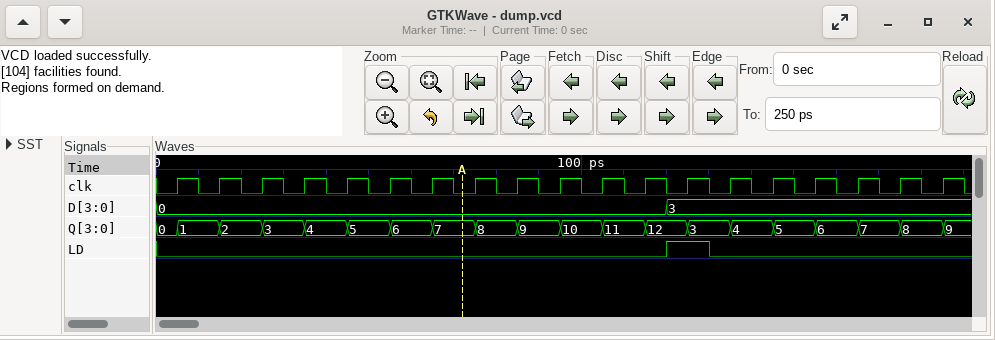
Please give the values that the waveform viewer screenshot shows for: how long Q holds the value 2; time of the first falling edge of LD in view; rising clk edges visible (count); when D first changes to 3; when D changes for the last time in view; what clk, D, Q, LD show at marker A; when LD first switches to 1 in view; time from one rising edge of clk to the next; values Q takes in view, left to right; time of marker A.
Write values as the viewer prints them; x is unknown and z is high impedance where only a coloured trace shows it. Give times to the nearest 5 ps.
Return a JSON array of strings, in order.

["10 ps", "130 ps", "19", "120 ps", "120 ps", "clk=0, D=0, Q=7, LD=0", "120 ps", "10 ps", "0, 1, 2, 3, 4, 5, 6, 7, 8, 9, 10, 11, 12, 3, 4, 5, 6, 7, 8, 9", "70 ps"]
